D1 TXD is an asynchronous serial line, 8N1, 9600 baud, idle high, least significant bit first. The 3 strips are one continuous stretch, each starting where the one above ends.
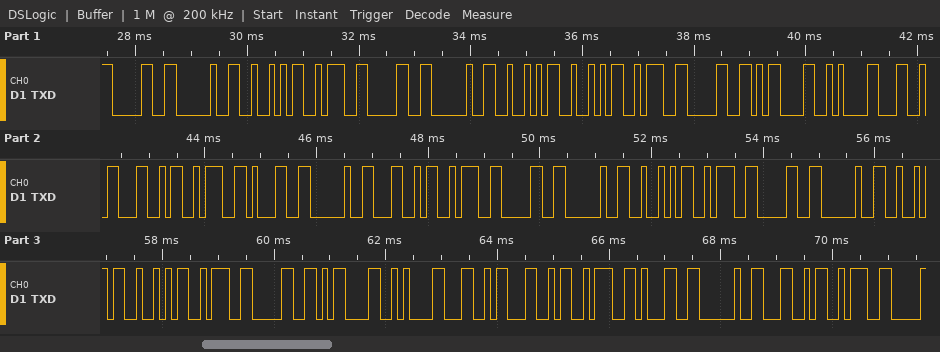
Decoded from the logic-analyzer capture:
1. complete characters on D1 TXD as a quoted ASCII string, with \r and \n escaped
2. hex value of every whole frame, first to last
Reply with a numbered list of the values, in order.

1. "0 R:0 RR:0\r\nLL:1 L:0 R:0 RR:0\r\nLL:1 L:"
2. 30 20 52 3A 30 20 52 52 3A 30 0D 0A 4C 4C 3A 31 20 4C 3A 30 20 52 3A 30 20 52 52 3A 30 0D 0A 4C 4C 3A 31 20 4C 3A
